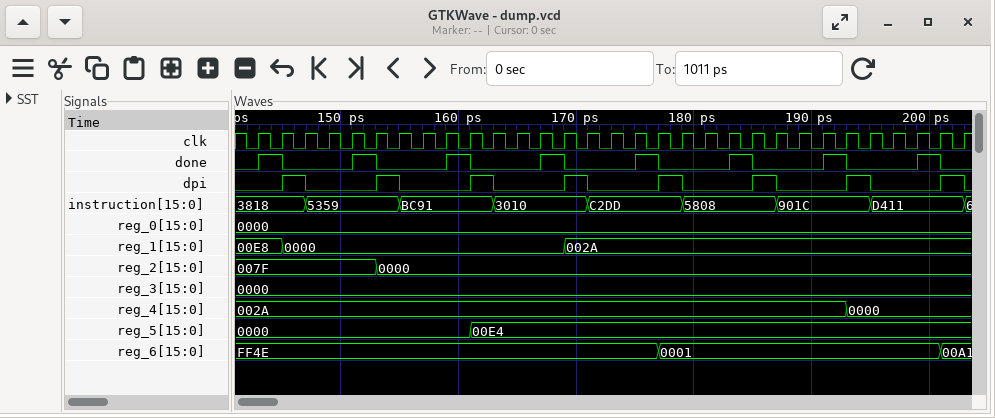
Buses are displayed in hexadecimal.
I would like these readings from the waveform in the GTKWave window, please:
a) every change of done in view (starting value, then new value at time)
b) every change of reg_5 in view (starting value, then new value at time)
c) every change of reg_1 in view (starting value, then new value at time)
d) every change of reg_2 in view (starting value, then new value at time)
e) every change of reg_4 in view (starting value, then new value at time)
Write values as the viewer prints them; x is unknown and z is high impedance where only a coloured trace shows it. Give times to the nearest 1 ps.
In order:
0, 1 at 143 ps, 0 at 145 ps, 1 at 151 ps, 0 at 153 ps, 1 at 159 ps, 0 at 161 ps, 1 at 167 ps, 0 at 169 ps, 1 at 175 ps, 0 at 177 ps, 1 at 183 ps, 0 at 185 ps, 1 at 191 ps, 0 at 193 ps, 1 at 199 ps, 0 at 201 ps
0000, 00E4 at 161 ps
00E8, 0000 at 145 ps, 002A at 169 ps
007F, 0000 at 153 ps
002A, 0000 at 193 ps
